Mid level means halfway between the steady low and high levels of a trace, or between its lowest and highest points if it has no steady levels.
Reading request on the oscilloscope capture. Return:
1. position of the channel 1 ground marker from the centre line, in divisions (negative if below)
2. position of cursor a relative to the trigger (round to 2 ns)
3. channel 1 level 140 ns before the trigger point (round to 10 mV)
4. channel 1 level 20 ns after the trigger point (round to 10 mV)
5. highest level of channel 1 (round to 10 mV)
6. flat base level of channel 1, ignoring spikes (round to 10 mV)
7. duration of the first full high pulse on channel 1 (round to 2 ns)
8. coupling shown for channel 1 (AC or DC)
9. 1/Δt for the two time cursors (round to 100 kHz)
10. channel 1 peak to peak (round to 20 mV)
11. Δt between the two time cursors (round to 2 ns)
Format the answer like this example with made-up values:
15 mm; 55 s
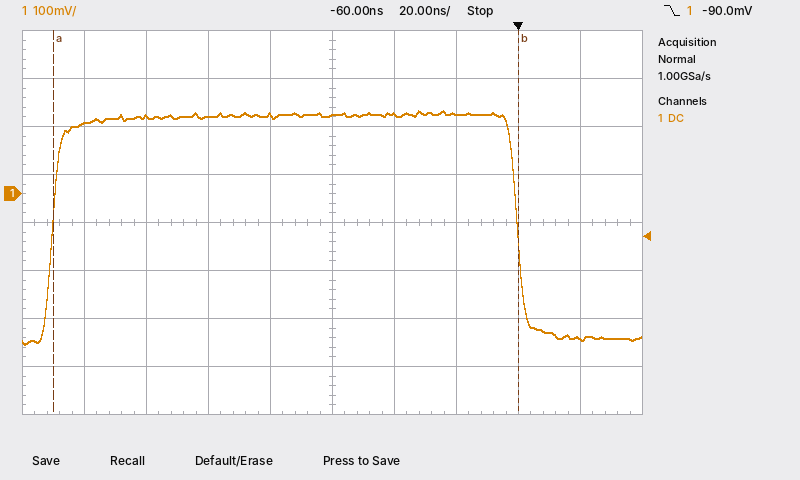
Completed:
+0.6 div; -150 ns; 150 mV; -300 mV; 170 mV; -300 mV; 150 ns; DC; 6.7 MHz; 480 mV; 150 ns
